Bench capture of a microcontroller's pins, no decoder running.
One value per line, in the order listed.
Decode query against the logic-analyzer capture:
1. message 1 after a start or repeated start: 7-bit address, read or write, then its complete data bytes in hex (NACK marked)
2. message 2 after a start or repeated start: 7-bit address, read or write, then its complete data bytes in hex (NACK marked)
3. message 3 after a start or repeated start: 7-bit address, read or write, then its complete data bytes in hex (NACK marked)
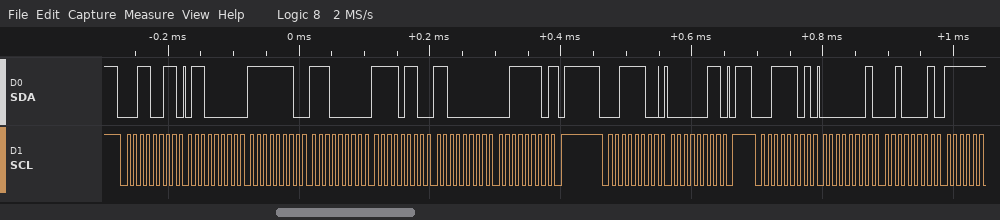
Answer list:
0x19 read: 60 FE E0 F6 C0 3E NACK
0x1E write: 03
0x1E read: 01 21
